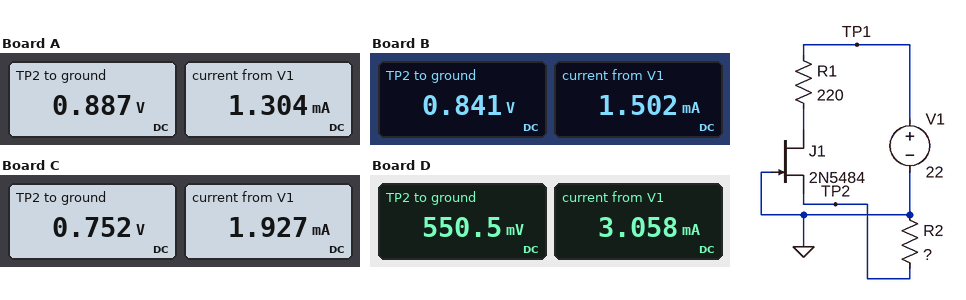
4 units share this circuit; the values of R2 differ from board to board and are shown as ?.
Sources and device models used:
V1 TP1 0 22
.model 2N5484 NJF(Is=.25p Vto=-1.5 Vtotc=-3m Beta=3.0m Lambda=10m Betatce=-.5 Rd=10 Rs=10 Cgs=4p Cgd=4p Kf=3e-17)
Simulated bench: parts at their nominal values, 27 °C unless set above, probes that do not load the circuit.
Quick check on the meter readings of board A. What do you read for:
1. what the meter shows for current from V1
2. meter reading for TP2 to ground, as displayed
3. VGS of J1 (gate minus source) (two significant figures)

1.304 mA
0.887 V
-890 mV
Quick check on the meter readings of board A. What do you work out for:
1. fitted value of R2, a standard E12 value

680 Ω
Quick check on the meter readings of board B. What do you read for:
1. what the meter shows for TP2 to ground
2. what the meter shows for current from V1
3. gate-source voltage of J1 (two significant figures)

0.841 V
1.502 mA
-840 mV
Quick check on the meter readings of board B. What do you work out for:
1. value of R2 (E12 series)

560 Ω
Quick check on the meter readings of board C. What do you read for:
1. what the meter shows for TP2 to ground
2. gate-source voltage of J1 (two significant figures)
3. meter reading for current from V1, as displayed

0.752 V
-750 mV
1.927 mA
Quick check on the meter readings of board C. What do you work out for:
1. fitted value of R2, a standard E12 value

390 Ω
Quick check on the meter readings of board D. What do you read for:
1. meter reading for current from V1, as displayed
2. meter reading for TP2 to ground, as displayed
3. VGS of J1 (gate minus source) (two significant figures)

3.058 mA
550.5 mV
-550 mV
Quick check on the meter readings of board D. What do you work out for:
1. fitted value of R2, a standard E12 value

180 Ω
